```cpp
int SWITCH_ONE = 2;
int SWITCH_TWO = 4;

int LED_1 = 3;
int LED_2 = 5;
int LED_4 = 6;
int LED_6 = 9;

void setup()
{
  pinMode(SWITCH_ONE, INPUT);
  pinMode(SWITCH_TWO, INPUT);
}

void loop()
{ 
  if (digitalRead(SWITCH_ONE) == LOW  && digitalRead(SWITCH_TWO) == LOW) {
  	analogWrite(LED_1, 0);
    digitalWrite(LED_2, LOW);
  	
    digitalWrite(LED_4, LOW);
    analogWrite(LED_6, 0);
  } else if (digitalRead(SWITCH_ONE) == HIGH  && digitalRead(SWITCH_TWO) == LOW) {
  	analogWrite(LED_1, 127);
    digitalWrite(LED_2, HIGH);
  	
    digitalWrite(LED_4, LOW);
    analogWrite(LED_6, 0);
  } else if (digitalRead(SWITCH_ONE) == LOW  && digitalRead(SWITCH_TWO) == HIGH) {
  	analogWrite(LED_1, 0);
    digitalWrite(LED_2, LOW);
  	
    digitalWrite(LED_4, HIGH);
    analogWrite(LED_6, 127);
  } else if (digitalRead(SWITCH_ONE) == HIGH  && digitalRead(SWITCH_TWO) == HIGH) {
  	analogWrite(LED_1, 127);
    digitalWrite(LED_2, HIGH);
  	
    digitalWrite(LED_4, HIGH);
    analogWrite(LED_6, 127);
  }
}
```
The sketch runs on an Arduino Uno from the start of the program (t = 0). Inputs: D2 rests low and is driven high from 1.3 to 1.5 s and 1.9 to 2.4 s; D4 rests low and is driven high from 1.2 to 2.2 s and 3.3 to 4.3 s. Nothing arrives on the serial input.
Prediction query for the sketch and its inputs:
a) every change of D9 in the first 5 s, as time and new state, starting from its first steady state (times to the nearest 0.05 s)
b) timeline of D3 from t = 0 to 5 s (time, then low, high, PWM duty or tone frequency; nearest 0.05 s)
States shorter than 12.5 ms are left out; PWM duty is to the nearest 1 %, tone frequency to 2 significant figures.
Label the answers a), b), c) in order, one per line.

a) 0 s low; 1.2 s PWM 50 %; 2.2 s low; 3.3 s PWM 50 %; 4.3 s low
b) 0 s low; 1.3 s PWM 50 %; 1.5 s low; 1.9 s PWM 50 %; 2.4 s low
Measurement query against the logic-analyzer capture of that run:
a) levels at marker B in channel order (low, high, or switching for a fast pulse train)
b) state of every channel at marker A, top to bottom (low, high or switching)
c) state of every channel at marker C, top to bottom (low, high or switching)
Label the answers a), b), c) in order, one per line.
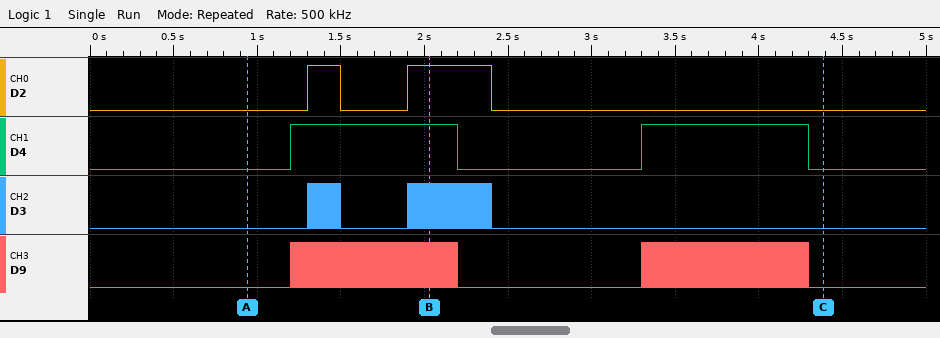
a) D2 high, D4 high, D3 switching, D9 switching
b) D2 low, D4 low, D3 low, D9 low
c) D2 low, D4 low, D3 low, D9 low
